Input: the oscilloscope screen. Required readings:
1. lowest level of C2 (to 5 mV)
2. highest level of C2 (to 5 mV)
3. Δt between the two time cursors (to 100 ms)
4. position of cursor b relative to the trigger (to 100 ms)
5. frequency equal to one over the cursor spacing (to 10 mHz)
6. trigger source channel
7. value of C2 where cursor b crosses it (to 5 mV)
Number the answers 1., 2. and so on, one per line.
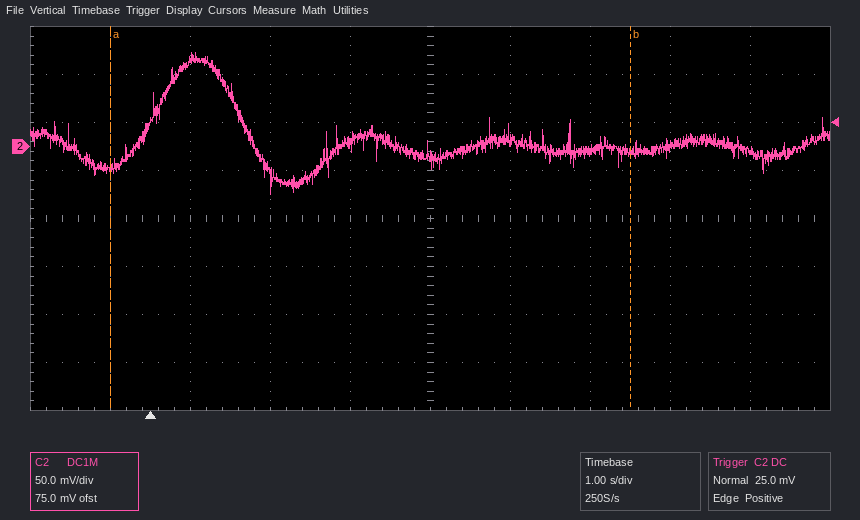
1. -50 mV
2. 100 mV
3. 6.5 s
4. +6.0 s
5. 150 mHz
6. C2
7. -5 mV
